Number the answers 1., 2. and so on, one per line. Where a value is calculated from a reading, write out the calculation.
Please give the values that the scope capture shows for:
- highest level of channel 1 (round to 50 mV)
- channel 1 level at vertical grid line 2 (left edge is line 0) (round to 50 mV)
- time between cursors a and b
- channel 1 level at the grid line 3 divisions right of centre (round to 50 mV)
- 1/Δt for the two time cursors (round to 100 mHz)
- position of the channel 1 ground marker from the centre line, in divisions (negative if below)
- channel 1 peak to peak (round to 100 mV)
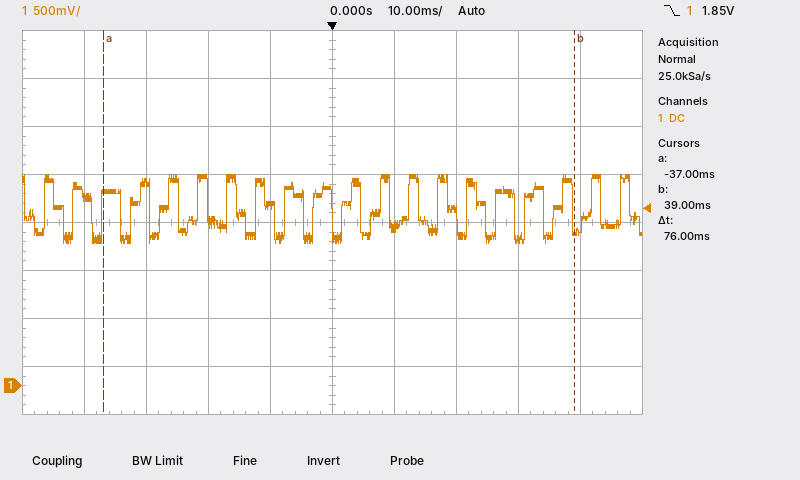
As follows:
1. 2.20 V
2. 2.10 V
3. 76 ms
4. 1.50 V
5. 1 / 76 ms ≈ 13.2 Hz
6. -3.4 div
7. 700 mV
